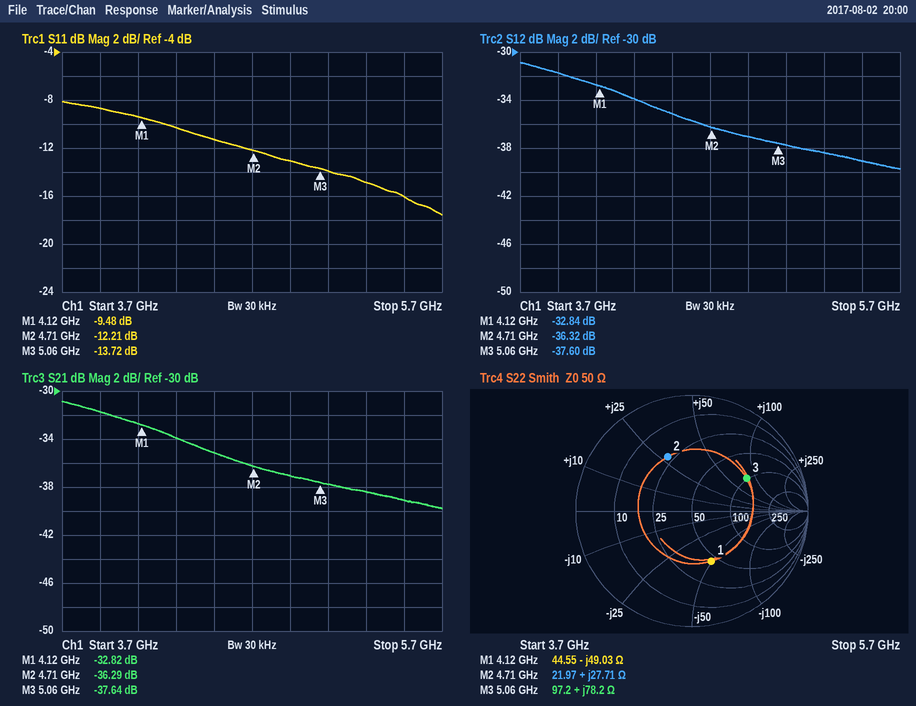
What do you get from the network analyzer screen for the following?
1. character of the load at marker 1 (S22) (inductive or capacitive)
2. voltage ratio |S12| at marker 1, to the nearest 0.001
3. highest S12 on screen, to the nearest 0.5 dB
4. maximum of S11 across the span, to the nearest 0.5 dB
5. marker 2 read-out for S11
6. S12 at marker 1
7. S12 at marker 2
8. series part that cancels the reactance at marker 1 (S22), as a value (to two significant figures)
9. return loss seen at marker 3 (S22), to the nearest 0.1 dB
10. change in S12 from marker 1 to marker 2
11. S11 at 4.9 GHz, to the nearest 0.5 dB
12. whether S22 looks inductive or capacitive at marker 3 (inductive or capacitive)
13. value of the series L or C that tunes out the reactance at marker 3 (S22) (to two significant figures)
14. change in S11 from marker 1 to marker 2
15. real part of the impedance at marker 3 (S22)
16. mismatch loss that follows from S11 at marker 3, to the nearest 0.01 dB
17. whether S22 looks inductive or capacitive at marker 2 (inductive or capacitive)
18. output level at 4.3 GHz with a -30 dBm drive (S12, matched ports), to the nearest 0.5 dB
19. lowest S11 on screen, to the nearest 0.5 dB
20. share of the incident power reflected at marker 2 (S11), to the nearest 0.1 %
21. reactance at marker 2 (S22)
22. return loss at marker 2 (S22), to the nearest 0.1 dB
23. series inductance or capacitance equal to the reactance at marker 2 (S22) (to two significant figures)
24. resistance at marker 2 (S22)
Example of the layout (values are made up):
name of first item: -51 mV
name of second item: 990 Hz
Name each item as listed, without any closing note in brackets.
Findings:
character of the load at marker 1 (S22): capacitive
voltage ratio |S12| at marker 1, to the nearest 0.001: 0.023
highest S12 on screen, to the nearest 0.5 dB: -31.0 dB
maximum of S11 across the span, to the nearest 0.5 dB: -8.0 dB
marker 2 read-out for S11: -12.21 dB
S12 at marker 1: -32.84 dB
S12 at marker 2: -36.32 dB
series part that cancels the reactance at marker 1 (S22), as a value: 1.9 nH
return loss seen at marker 3 (S22), to the nearest 0.1 dB: 5.2 dB
change in S12 from marker 1 to marker 2: -3.48 dB
S11 at 4.9 GHz, to the nearest 0.5 dB: -13.0 dB
whether S22 looks inductive or capacitive at marker 3: inductive
value of the series L or C that tunes out the reactance at marker 3 (S22): 400 fF
change in S11 from marker 1 to marker 2: -2.73 dB
real part of the impedance at marker 3: 97.2 Ω
mismatch loss that follows from S11 at marker 3, to the nearest 0.01 dB: 0.19 dB
whether S22 looks inductive or capacitive at marker 2: inductive
output level at 4.3 GHz with a -30 dBm drive (S12, matched ports), to the nearest 0.5 dB: -64.0 dBm
lowest S11 on screen, to the nearest 0.5 dB: -17.5 dB
share of the incident power reflected at marker 2 (S11), to the nearest 0.1 %: 6.0 %
reactance at marker 2: +27.71 Ω
return loss at marker 2 (S22), to the nearest 0.1 dB: 5.8 dB
series inductance or capacitance equal to the reactance at marker 2 (S22): 940 pH
resistance at marker 2: 21.97 Ω
